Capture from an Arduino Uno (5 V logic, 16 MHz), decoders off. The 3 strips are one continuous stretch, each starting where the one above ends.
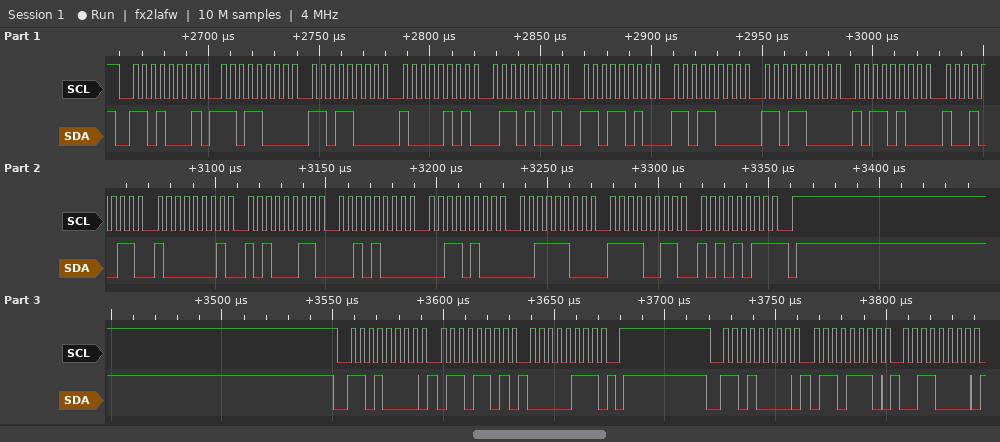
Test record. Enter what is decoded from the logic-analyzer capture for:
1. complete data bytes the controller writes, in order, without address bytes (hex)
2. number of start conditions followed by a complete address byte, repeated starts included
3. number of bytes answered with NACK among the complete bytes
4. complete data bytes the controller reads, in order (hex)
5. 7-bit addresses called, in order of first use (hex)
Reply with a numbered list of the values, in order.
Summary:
1. 6D 07 6E 30
2. 3
3. 1
4. D8 D8 85 69 DA D8 D8 B4 93 81 A3 28 34 3C F3 AB
5. 0x68
